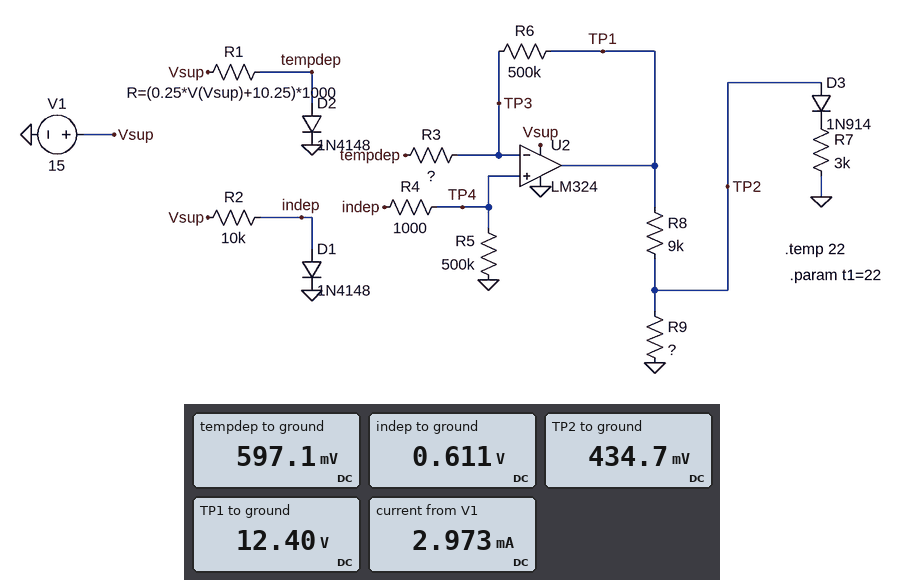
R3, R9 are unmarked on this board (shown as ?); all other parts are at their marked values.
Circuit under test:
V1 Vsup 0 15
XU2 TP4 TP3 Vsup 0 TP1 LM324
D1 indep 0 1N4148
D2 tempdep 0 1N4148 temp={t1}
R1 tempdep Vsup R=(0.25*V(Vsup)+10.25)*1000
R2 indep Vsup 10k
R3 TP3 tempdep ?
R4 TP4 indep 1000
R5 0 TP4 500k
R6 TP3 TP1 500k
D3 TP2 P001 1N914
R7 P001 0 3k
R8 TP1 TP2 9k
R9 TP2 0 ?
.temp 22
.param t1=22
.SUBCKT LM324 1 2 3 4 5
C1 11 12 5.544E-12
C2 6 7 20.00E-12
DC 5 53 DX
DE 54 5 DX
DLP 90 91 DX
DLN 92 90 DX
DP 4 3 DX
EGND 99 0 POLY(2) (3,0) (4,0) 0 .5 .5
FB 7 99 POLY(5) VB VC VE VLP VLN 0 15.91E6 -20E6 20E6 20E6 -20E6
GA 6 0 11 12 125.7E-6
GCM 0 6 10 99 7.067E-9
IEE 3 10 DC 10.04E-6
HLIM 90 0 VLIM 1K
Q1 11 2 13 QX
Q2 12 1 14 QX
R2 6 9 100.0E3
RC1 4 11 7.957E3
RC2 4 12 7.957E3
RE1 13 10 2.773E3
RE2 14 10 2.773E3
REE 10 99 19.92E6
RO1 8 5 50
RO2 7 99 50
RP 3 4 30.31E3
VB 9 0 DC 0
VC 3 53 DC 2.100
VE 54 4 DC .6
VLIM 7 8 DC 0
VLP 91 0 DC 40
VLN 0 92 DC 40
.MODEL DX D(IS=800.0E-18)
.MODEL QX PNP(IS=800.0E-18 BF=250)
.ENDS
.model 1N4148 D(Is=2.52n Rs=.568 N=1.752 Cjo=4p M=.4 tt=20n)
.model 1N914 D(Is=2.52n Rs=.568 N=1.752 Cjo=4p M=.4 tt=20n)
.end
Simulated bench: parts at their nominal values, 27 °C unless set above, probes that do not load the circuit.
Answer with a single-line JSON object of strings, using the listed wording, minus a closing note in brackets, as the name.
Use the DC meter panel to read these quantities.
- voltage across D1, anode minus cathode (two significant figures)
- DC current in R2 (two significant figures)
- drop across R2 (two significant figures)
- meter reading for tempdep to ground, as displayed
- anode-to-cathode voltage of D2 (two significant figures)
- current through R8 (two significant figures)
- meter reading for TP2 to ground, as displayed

{"voltage across D1, anode minus cathode": "610 mV", "DC current in R2": "1.4 mA", "drop across R2": "14 V", "meter reading for tempdep to ground, as displayed": "597.1 mV", "anode-to-cathode voltage of D2": "600 mV", "current through R8": "1.3 mA", "meter reading for TP2 to ground, as displayed": "434.7 mV"}
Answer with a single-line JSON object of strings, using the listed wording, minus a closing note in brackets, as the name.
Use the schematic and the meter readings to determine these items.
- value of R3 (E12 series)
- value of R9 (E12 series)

{"value of R3": "560 Ω", "value of R9": "330 Ω"}
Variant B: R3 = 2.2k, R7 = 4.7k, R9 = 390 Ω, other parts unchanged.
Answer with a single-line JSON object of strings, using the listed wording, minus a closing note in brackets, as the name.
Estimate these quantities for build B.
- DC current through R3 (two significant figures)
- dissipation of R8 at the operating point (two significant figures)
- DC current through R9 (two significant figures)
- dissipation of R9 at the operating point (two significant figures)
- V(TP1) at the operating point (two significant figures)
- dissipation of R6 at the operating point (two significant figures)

{"DC current through R3": "6.4 µA", "dissipation of R8 at the operating point": "1.5 mW", "DC current through R9": "400 µA", "dissipation of R9 at the operating point": "64 µW", "V(TP1) at the operating point": "3.8 V", "dissipation of R6 at the operating point": "20 µW"}
